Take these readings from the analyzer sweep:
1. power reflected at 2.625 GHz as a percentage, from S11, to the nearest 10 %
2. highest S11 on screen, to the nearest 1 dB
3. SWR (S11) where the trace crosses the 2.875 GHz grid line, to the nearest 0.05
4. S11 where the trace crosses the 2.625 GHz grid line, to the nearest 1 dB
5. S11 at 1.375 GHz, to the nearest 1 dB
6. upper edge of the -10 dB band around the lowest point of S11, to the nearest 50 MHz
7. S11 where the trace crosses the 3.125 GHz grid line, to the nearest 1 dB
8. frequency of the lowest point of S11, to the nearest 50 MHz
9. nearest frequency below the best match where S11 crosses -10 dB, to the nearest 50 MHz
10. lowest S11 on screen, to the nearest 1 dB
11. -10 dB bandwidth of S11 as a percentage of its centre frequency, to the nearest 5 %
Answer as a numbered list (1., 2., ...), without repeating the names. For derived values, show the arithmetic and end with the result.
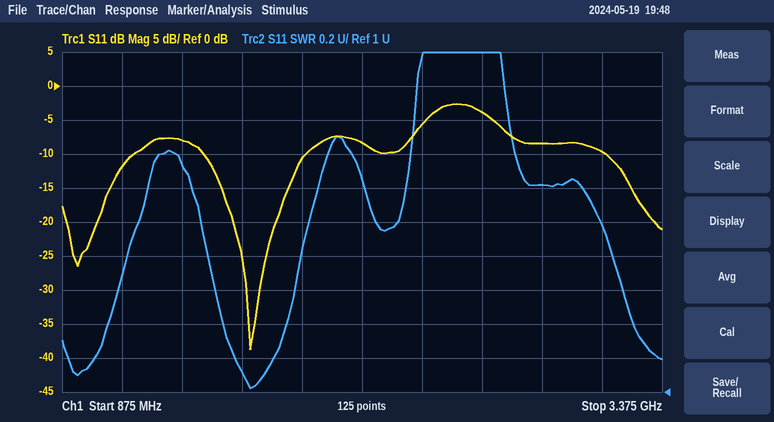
1. 10^(-4/10) ≈ 40 %
2. -3 dB
3. 2.20
4. -4 dB
5. -8 dB
6. 1.90 GHz
7. -10 dB
8. 1.65 GHz
9. 1.45 GHz
10. -39 dB
11. 450 MHz / 1.675 GHz ≈ 26.9 %, so 25 % to the nearest 5 %
